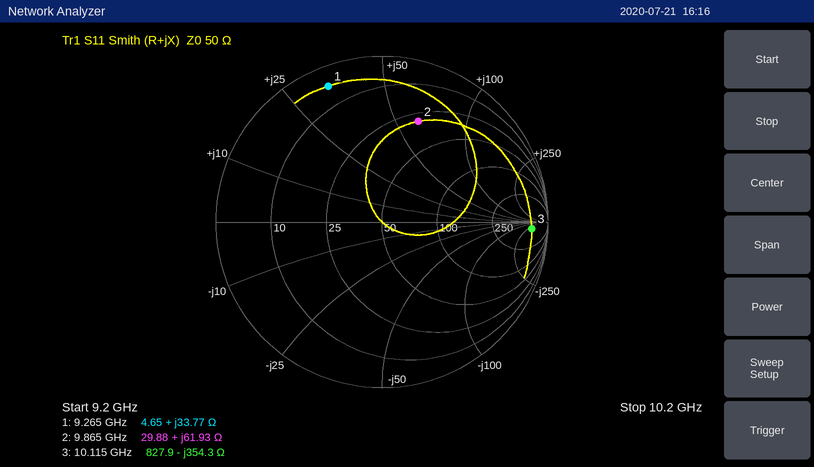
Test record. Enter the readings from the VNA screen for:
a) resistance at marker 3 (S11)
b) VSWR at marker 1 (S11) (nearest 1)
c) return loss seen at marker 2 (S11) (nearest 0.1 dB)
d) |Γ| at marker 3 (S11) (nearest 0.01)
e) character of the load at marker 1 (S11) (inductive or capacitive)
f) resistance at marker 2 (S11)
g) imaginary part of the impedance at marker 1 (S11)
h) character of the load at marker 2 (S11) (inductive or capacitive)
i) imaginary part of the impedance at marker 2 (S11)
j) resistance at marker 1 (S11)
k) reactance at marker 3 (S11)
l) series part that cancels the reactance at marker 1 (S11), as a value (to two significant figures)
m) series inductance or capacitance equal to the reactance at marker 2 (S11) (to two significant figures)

827.9 Ω
16
3.8 dB
0.90
inductive
29.88 Ω
+33.77 Ω
inductive
+61.93 Ω
4.65 Ω
-354.3 Ω
510 fF
1.00 nH
